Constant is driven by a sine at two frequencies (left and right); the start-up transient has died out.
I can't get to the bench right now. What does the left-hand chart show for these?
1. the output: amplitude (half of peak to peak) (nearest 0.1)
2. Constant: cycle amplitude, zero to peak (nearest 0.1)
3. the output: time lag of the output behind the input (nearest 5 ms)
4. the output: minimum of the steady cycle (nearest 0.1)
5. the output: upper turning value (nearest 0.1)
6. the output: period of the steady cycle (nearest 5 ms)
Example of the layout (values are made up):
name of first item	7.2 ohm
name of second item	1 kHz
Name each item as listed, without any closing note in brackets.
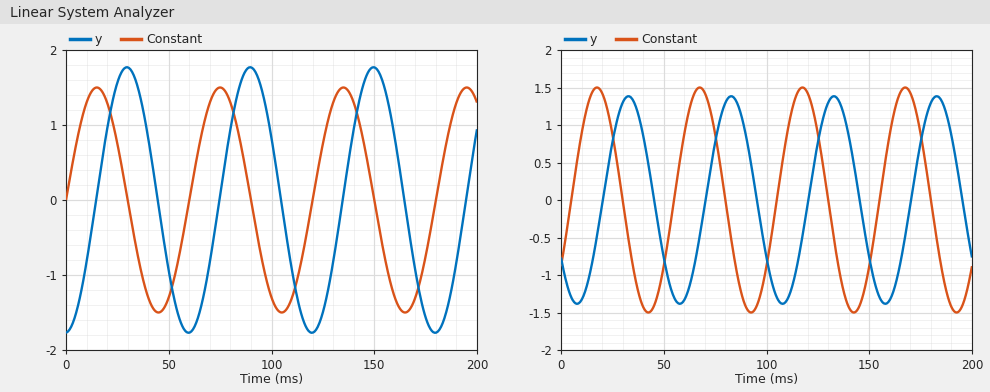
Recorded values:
the output: amplitude (half of peak to peak)	1.8
Constant: cycle amplitude, zero to peak	1.5
the output: time lag of the output behind the input	15 ms
the output: minimum of the steady cycle	-1.8
the output: upper turning value	1.8
the output: period of the steady cycle	60 ms
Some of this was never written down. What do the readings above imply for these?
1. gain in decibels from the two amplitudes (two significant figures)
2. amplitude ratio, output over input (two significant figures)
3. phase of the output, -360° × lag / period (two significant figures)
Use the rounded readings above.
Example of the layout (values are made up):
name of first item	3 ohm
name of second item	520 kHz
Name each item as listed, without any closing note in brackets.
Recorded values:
gain in decibels from the two amplitudes	1.6 dB
amplitude ratio, output over input	1.2
phase of the output, -360° × lag / period	-90°
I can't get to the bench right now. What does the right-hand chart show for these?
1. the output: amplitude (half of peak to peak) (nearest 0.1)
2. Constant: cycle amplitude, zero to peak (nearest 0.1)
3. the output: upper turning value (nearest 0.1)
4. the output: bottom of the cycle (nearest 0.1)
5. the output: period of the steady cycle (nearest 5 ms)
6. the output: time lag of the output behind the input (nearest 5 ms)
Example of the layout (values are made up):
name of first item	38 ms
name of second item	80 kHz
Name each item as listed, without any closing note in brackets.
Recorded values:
the output: amplitude (half of peak to peak)	1.4
Constant: cycle amplitude, zero to peak	1.5
the output: upper turning value	1.4
the output: bottom of the cycle	-1.4
the output: period of the steady cycle	50 ms
the output: time lag of the output behind the input	15 ms
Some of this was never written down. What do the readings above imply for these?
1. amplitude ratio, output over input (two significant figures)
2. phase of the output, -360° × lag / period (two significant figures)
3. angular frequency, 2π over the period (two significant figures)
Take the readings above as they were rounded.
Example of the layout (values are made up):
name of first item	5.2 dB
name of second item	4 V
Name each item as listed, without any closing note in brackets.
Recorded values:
amplitude ratio, output over input	0.93
phase of the output, -360° × lag / period	-110°
angular frequency, 2π over the period	0.13 rad/ms
